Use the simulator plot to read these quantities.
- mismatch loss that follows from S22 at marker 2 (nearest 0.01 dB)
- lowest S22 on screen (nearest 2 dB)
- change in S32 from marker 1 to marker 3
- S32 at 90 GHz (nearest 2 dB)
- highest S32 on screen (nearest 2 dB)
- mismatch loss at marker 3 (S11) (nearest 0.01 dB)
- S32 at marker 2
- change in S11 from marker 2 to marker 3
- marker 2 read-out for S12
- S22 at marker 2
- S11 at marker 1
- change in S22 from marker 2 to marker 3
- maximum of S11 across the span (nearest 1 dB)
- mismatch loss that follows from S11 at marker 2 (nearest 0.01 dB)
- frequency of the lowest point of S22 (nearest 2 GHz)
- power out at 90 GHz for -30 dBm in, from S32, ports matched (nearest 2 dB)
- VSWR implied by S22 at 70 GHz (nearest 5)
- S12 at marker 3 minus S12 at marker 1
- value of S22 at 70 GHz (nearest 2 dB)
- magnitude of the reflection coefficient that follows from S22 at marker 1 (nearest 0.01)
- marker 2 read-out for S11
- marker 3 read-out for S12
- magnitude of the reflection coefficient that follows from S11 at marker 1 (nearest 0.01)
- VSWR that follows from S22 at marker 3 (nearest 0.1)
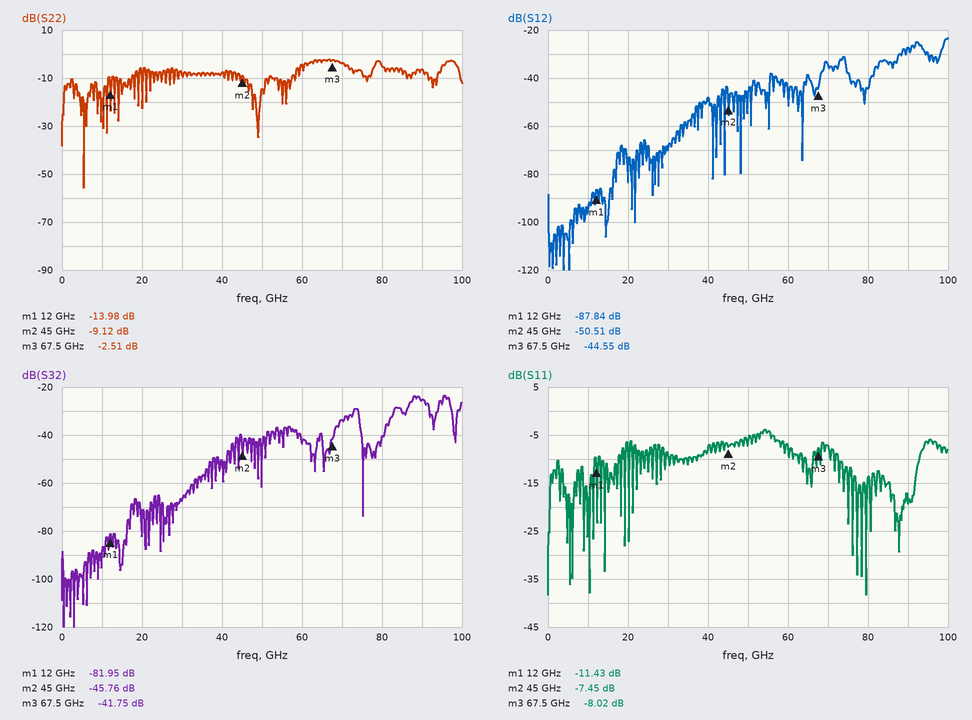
0.57 dB
-56 dB
40.20 dB
-26 dB
-24 dB
0.75 dB
-45.76 dB
-0.57 dB
-50.51 dB
-9.12 dB
-11.43 dB
6.61 dB
-4 dB
0.86 dB
6 GHz
-56 dBm
5
43.29 dB
-4 dB
0.20
-7.45 dB
-44.55 dB
0.27
7.0
